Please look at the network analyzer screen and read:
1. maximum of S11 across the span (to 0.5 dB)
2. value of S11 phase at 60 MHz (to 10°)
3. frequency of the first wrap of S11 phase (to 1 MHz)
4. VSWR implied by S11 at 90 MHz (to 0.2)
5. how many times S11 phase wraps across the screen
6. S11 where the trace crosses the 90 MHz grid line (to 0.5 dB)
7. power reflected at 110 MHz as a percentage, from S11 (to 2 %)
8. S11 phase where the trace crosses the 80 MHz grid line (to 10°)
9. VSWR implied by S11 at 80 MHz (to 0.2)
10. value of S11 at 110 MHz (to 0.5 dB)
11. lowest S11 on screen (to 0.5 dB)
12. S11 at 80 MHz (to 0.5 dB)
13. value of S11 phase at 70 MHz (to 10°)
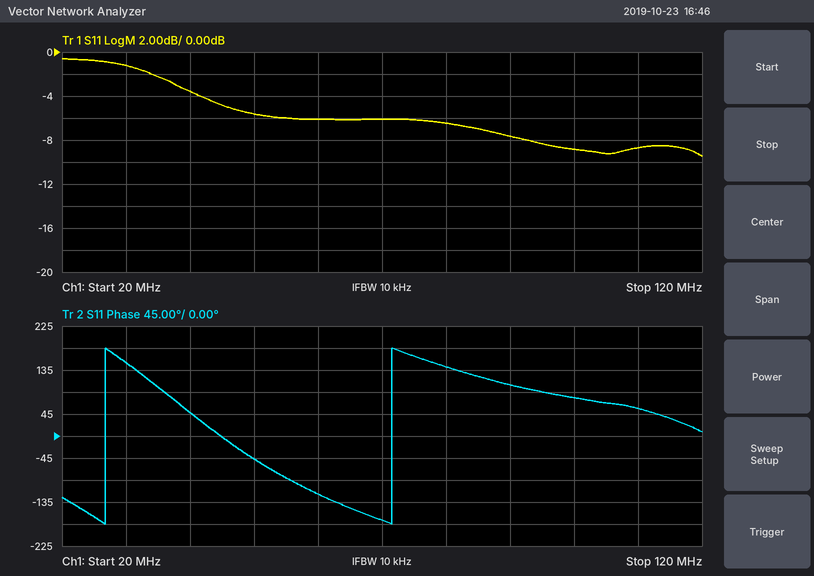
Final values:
-0.5 dB
-120°
27 MHz
2.4
2
-7.5 dB
14 %
140°
2.8
-8.5 dB
-9.5 dB
-6.5 dB
-170°
